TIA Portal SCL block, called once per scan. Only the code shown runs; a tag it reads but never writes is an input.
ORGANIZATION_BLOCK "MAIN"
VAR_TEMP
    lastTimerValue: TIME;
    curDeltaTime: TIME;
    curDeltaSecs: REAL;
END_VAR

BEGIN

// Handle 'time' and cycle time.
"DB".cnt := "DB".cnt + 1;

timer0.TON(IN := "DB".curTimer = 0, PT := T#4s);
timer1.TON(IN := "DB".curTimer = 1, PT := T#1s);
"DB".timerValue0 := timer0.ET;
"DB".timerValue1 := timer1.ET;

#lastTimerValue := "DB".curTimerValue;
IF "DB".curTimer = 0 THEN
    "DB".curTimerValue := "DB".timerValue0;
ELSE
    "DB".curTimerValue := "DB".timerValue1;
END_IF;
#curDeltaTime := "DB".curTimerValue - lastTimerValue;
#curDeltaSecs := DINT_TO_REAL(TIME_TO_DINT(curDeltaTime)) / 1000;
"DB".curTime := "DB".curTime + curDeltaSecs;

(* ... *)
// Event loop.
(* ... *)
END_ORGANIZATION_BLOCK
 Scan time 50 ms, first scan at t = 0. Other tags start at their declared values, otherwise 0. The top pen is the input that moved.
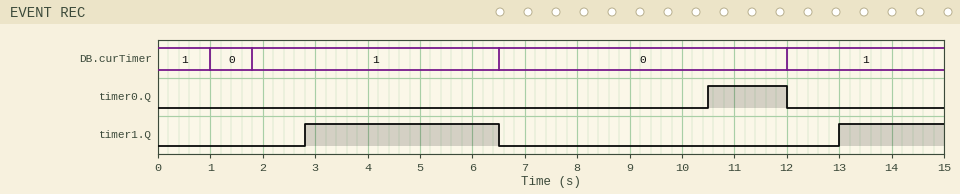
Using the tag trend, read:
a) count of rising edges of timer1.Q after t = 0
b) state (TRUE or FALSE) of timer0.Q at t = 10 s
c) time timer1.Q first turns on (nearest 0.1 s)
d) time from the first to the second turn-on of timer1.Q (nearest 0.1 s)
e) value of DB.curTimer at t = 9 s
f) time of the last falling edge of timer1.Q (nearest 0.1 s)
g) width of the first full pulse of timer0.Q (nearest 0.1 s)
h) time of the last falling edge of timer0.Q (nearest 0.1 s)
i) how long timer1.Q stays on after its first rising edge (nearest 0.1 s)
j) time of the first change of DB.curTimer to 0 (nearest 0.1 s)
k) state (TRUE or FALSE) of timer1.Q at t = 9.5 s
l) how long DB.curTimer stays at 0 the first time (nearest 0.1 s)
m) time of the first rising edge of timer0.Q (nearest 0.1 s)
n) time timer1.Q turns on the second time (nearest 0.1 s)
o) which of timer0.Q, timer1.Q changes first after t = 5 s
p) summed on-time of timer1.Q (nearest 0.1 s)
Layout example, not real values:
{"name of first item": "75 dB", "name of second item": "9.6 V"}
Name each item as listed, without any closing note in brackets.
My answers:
{"count of rising edges of timer1.Q after t = 0": "2", "state (TRUE or FALSE) of timer0.Q at t = 10 s": "FALSE", "time timer1.Q first turns on": "2.8 s", "time from the first to the second turn-on of timer1.Q": "10.2 s", "value of DB.curTimer at t = 9 s": "0", "time of the last falling edge of timer1.Q": "6.5 s", "width of the first full pulse of timer0.Q": "1.5 s", "time of the last falling edge of timer0.Q": "12.0 s", "how long timer1.Q stays on after its first rising edge": "3.7 s", "time of the first change of DB.curTimer to 0": "1.0 s", "state (TRUE or FALSE) of timer1.Q at t = 9.5 s": "FALSE", "how long DB.curTimer stays at 0 the first time": "0.8 s", "time of the first rising edge of timer0.Q": "10.5 s", "time timer1.Q turns on the second time": "13.0 s", "which of timer0.Q, timer1.Q changes first after t = 5 s": "timer1.Q", "summed on-time of timer1.Q": "5.7 s"}
